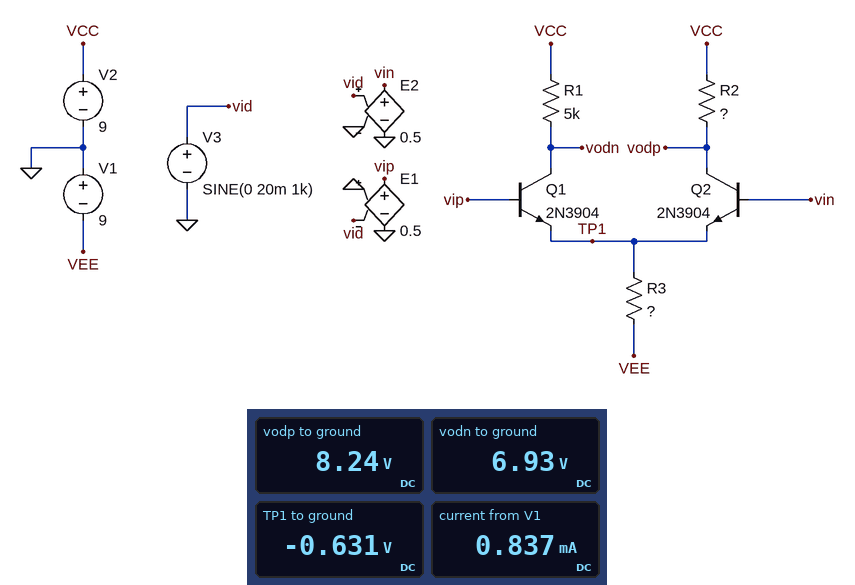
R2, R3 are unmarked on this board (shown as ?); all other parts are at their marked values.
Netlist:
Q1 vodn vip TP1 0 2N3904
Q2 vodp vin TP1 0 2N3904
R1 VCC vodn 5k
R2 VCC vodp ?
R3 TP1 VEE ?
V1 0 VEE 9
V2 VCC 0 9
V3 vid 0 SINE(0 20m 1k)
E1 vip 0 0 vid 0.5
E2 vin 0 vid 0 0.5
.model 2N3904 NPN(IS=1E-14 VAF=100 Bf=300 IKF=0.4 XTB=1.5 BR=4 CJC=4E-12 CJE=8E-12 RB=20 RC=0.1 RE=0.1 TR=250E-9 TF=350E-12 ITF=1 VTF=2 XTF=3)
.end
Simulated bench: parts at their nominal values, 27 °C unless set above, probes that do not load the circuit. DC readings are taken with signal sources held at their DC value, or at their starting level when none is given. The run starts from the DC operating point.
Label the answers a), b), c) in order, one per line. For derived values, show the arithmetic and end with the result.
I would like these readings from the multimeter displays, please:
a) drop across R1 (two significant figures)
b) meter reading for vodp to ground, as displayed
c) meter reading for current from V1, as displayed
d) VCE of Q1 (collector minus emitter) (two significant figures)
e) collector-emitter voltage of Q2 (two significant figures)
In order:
a) 9 V - 6.93 V = 2.1 V
b) 8.24 V
c) 0.837 mA
d) 6.93 V - (-631 mV) = 7.6 V
e) 8.24 V - (-631 mV) = 8.9 V
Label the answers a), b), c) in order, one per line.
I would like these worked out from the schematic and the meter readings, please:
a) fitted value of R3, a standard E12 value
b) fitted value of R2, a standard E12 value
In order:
a) 10 kΩ
b) 1.8 kΩ
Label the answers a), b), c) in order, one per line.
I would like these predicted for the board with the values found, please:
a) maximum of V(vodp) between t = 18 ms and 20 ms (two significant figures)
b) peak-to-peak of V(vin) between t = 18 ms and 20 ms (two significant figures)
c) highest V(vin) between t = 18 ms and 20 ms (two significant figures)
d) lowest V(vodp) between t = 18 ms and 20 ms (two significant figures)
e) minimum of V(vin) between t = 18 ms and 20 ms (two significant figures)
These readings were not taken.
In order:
a) 8.5 V
b) 20 mV
c) 10 mV
d) 8.0 V
e) -10 mV
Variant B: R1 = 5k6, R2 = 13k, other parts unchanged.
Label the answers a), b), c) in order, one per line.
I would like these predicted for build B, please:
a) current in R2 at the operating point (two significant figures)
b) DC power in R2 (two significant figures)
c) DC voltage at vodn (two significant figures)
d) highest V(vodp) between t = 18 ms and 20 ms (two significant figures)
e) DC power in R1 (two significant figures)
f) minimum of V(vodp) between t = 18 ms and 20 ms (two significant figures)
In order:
a) 410 µA
b) 2.2 mW
c) 6.6 V
d) 5.6 V
e) 1.0 mW
f) 1.7 V
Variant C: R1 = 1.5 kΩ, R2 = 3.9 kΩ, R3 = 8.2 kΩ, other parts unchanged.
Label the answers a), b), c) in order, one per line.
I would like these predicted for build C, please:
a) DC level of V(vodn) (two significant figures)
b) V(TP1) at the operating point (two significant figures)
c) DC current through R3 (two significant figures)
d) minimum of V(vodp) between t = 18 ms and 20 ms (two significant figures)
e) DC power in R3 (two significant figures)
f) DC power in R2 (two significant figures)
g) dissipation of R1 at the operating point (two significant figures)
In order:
a) 8.2 V
b) -640 mV
c) 1.0 mA
d) 6.3 V
e) 8.5 mW
f) 1.0 mW
g) 390 µW
